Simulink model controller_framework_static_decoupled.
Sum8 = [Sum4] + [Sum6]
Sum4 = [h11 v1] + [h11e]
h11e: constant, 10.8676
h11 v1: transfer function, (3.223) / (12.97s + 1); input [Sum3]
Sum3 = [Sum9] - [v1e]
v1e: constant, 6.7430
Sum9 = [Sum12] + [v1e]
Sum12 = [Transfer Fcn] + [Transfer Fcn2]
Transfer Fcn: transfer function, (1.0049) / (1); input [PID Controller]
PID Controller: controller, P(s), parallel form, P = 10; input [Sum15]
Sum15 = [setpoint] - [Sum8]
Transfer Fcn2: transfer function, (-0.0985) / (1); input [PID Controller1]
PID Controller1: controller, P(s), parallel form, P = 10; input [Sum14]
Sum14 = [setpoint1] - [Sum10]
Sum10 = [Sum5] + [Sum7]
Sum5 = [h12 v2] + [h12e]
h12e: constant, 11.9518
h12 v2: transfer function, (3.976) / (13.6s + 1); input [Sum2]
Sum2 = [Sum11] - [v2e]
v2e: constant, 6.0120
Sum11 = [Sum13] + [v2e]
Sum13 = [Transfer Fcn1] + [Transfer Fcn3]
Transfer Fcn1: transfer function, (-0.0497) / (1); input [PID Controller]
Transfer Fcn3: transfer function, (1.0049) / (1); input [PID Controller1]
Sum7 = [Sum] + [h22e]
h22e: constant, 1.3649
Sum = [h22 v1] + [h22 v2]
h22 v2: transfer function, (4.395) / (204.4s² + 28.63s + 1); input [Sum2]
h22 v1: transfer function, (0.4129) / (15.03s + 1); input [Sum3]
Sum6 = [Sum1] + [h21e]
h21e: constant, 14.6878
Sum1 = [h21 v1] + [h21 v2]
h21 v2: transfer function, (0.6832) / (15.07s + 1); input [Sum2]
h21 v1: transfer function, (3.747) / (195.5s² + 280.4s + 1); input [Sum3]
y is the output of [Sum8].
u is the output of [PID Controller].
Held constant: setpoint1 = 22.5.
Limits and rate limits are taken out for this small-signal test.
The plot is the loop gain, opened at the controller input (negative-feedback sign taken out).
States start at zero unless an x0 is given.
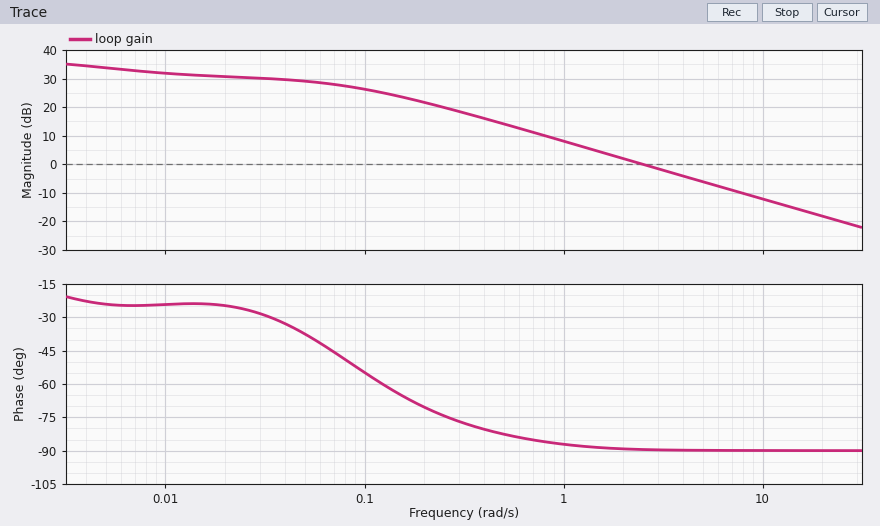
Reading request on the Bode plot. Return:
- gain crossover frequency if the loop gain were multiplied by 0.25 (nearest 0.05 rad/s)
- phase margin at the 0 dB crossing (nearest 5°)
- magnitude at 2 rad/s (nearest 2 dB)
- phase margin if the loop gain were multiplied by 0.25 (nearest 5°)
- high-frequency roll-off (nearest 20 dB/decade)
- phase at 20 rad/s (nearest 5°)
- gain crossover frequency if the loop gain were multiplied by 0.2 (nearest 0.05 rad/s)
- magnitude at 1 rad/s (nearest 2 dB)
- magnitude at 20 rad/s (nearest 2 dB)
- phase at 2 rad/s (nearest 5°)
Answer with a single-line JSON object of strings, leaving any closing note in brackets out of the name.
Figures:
{"gain crossover frequency if the loop gain were multiplied by 0.25": "0.65 rad/s", "phase margin at the 0 dB crossing": "90°", "magnitude at 2 rad/s": "2 dB", "phase margin if the loop gain were multiplied by 0.25": "95°", "high-frequency roll-off": "-20 dB/decade", "phase at 20 rad/s": "-90°", "gain crossover frequency if the loop gain were multiplied by 0.2": "0.50 rad/s", "magnitude at 1 rad/s": "8 dB", "magnitude at 20 rad/s": "-18 dB", "phase at 2 rad/s": "-90°"}
